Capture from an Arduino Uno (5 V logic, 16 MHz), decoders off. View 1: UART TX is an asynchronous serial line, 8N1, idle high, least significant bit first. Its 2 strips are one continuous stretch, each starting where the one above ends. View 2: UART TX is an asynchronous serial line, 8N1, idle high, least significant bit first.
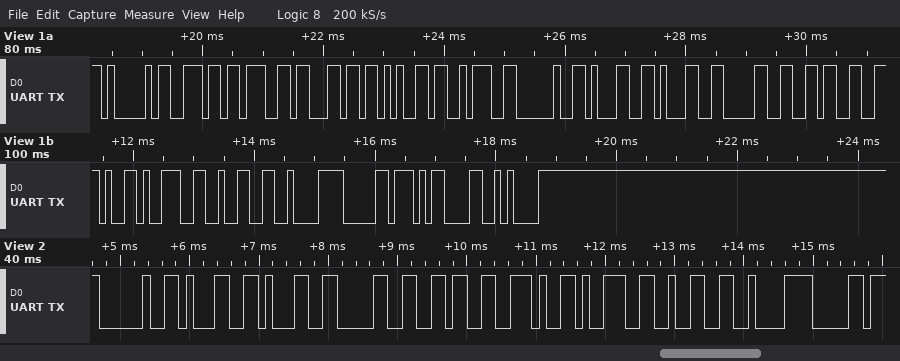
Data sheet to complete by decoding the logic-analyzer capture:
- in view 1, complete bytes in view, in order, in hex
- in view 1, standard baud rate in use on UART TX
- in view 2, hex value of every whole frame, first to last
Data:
41 6E 67 6C 65 3A 20 31 31 30 36 2E 39 32 C2 B0 0D 0A
9600 baud
20 31 31 30 36 2E 39 32 C2 B0
